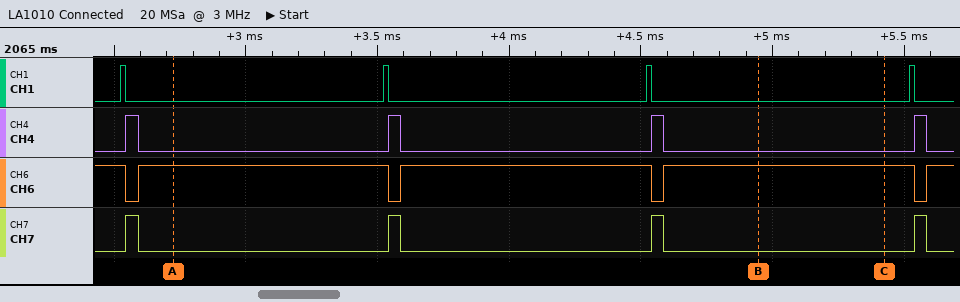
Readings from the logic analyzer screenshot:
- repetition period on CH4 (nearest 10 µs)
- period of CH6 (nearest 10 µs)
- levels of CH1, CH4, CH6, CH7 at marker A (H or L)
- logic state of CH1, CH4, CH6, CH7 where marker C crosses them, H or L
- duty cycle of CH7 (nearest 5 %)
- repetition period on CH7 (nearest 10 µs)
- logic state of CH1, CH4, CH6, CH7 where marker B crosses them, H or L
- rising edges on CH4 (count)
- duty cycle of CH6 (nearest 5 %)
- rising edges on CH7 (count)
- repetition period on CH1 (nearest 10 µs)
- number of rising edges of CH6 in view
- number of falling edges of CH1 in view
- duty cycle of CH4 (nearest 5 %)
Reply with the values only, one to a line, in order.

1000 µs
1000 µs
CH1=L, CH4=L, CH6=H, CH7=L
CH1=L, CH4=L, CH6=H, CH7=L
5 %
1000 µs
CH1=L, CH4=L, CH6=H, CH7=L
4
95 %
4
1000 µs
4
4
5 %
